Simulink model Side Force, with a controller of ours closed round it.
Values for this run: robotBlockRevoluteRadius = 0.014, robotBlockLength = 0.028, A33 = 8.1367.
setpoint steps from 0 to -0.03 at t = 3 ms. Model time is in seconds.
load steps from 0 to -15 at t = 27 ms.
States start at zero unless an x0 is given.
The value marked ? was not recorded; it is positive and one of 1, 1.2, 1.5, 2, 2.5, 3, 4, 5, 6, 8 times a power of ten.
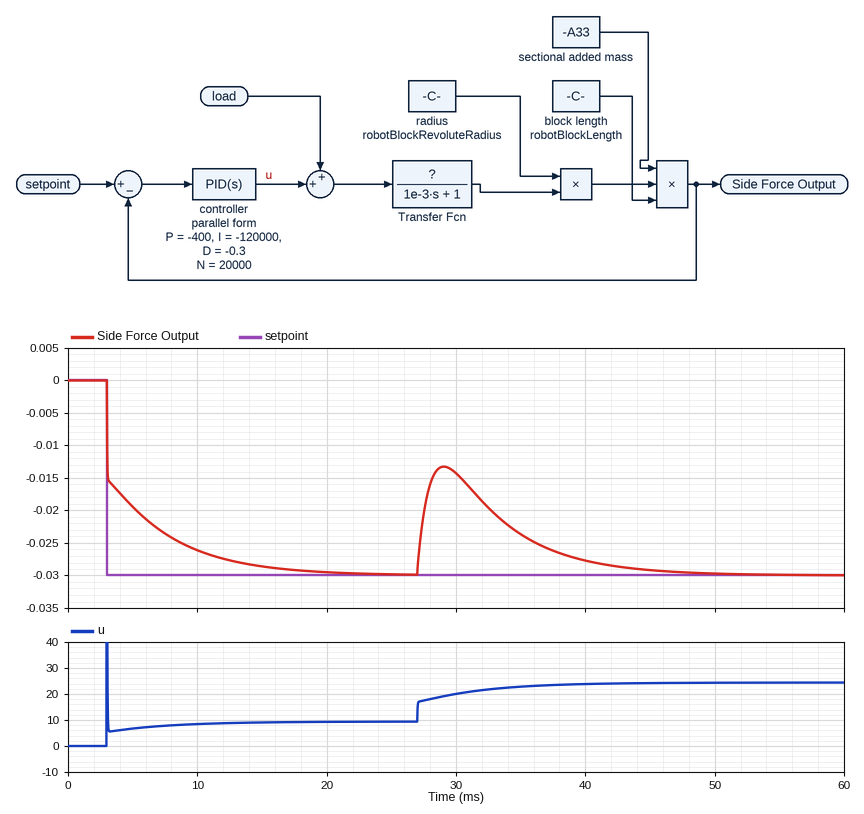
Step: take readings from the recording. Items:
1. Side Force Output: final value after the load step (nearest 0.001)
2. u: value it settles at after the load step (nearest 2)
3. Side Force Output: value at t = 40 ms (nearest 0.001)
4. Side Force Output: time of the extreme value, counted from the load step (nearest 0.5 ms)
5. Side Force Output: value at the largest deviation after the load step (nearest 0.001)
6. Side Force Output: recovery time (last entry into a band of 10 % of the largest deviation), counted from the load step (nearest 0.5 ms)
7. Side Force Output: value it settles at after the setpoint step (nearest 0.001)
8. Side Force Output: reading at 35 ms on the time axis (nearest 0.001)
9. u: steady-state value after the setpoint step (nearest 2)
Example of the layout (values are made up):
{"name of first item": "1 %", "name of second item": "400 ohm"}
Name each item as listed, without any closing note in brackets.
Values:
{"Side Force Output: final value after the load step": "-0.030", "u: value it settles at after the load step": "24", "Side Force Output: value at t = 40 ms": "-0.028", "Side Force Output: time of the extreme value, counted from the load step": "2.0 ms", "Side Force Output: value at the largest deviation after the load step": "-0.013", "Side Force Output: recovery time (last entry into a band of 10 % of the largest deviation), counted from the load step": "14.5 ms", "Side Force Output: value it settles at after the setpoint step": "-0.030", "Side Force Output: reading at 35 ms on the time axis": "-0.024", "u: steady-state value after the setpoint step": "10"}
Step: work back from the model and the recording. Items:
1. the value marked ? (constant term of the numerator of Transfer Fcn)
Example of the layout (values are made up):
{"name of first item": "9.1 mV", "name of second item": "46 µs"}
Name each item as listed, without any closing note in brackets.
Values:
{"the value marked ?": "1"}
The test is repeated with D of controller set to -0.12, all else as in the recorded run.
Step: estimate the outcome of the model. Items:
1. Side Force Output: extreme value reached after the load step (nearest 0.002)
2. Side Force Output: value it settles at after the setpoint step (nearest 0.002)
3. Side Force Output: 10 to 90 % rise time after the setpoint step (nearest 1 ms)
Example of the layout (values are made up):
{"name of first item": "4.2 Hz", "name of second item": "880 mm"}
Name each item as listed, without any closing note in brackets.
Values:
{"Side Force Output: extreme value reached after the load step": "-0.012", "Side Force Output: value it settles at after the setpoint step": "-0.030", "Side Force Output: 10 to 90 % rise time after the setpoint step": "8 ms"}
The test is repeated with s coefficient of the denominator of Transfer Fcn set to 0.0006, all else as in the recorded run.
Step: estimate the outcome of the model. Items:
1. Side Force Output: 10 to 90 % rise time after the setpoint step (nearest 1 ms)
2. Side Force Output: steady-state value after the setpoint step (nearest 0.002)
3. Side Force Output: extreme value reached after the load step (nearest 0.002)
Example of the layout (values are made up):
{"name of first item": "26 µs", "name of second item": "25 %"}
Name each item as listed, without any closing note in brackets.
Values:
{"Side Force Output: 10 to 90 % rise time after the setpoint step": "9 ms", "Side Force Output: steady-state value after the setpoint step": "-0.030", "Side Force Output: extreme value reached after the load step": "-0.012"}
